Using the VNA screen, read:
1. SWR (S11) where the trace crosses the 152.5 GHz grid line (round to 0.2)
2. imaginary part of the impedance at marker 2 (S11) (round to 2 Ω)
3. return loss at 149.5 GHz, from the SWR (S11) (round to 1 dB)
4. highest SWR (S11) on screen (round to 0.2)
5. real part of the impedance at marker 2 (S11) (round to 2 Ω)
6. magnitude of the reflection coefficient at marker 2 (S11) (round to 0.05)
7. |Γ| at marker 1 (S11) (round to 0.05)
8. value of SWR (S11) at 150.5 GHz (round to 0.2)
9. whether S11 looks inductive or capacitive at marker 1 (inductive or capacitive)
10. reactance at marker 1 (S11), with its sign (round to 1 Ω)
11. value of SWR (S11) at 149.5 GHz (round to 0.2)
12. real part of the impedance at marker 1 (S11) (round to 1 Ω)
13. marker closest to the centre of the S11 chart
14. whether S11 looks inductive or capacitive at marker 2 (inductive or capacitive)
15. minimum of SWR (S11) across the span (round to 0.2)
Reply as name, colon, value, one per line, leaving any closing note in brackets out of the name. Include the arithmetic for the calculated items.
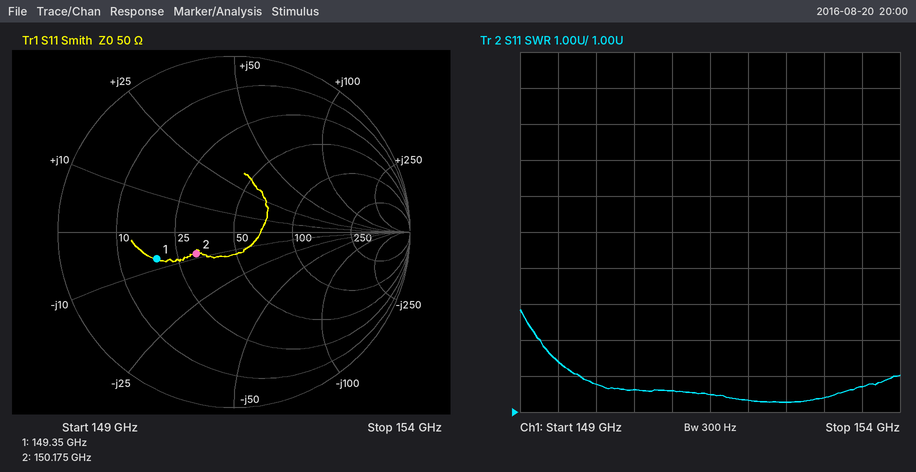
SWR (S11) where the trace crosses the 152.5 GHz grid line: 1.2
imaginary part of the impedance at marker 2 (S11): -8 Ω
return loss at 149.5 GHz, from the SWR (S11): −20 log10((2.4 − 1)/(2.4 + 1)) ≈ 8 dB
highest SWR (S11) on screen: 3.8
real part of the impedance at marker 2 (S11): 32 Ω
magnitude of the reflection coefficient at marker 2 (S11): 0.25
|Γ| at marker 1 (S11): 0.45
value of SWR (S11) at 150.5 GHz: 1.6
whether S11 looks inductive or capacitive at marker 1: capacitive
reactance at marker 1 (S11), with its sign: -7 Ω
value of SWR (S11) at 149.5 GHz: 2.4
real part of the impedance at marker 1 (S11): 19 Ω
marker closest to the centre of the S11 chart: marker 2
whether S11 looks inductive or capacitive at marker 2: capacitive
minimum of SWR (S11) across the span: 1.2
